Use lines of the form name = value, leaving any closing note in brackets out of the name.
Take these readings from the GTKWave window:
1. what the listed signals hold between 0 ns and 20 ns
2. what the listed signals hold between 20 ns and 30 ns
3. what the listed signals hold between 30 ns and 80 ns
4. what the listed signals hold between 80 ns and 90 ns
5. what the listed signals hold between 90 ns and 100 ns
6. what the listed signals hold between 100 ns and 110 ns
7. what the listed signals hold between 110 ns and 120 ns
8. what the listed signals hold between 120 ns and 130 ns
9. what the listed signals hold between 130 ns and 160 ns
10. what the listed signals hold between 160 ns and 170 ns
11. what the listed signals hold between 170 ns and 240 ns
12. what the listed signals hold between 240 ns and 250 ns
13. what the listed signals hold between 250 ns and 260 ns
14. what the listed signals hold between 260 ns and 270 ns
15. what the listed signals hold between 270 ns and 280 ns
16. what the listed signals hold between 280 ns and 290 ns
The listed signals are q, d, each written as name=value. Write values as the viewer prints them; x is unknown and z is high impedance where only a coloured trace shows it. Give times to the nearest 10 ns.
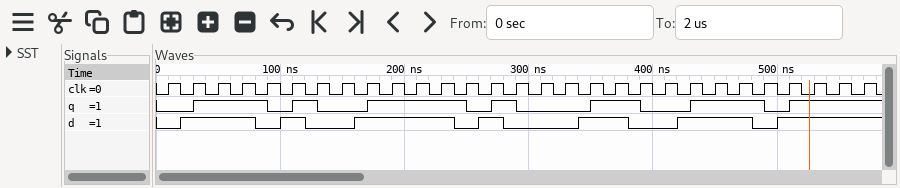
what the listed signals hold between 0 ns and 20 ns = q=0, d=0
what the listed signals hold between 20 ns and 30 ns = q=0, d=1
what the listed signals hold between 30 ns and 80 ns = q=1, d=1
what the listed signals hold between 80 ns and 90 ns = q=1, d=0
what the listed signals hold between 90 ns and 100 ns = q=0, d=0
what the listed signals hold between 100 ns and 110 ns = q=0, d=1
what the listed signals hold between 110 ns and 120 ns = q=1, d=1
what the listed signals hold between 120 ns and 130 ns = q=1, d=0
what the listed signals hold between 130 ns and 160 ns = q=0, d=0
what the listed signals hold between 160 ns and 170 ns = q=0, d=1
what the listed signals hold between 170 ns and 240 ns = q=1, d=1
what the listed signals hold between 240 ns and 250 ns = q=1, d=0
what the listed signals hold between 250 ns and 260 ns = q=0, d=0
what the listed signals hold between 260 ns and 270 ns = q=0, d=1
what the listed signals hold between 270 ns and 280 ns = q=1, d=1
what the listed signals hold between 280 ns and 290 ns = q=1, d=0
